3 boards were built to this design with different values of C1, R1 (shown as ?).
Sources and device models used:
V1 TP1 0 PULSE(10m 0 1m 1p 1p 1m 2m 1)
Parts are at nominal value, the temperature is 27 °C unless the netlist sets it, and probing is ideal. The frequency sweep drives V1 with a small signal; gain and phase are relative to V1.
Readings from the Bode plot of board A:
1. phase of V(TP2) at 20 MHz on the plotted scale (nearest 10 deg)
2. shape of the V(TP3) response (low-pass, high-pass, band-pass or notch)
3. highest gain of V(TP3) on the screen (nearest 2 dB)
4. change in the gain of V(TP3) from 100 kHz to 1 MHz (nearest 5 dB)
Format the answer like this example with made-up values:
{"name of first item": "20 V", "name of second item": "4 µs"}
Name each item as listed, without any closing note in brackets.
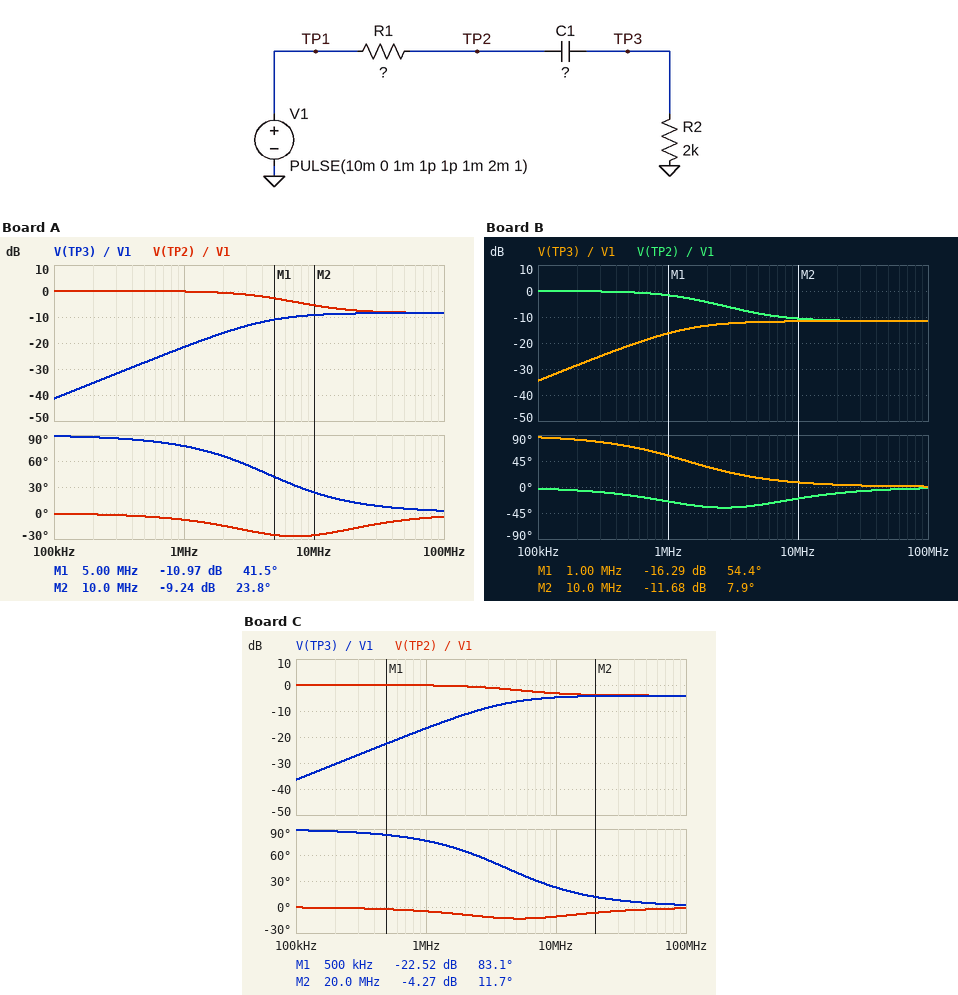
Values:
{"phase of V(TP2) at 20 MHz on the plotted scale": "-20 deg", "shape of the V(TP3) response": "high-pass", "highest gain of V(TP3) on the screen": "-8 dB", "change in the gain of V(TP3) from 100 kHz to 1 MHz": "20 dB"}
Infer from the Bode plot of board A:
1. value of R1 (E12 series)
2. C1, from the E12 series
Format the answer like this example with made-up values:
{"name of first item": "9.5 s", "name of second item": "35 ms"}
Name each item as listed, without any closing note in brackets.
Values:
{"value of R1": "3.3 kΩ", "C1, from the E12 series": "6.8 pF"}
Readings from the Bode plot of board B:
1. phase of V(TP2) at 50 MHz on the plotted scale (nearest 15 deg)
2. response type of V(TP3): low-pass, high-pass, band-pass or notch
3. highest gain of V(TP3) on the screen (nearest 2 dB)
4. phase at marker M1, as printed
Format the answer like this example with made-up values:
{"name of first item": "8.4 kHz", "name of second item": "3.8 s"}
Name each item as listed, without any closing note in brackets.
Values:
{"phase of V(TP2) at 50 MHz on the plotted scale": "0 deg", "response type of V(TP3): low-pass, high-pass, band-pass or notch": "high-pass", "highest gain of V(TP3) on the screen": "-12 dB", "phase at marker M1, as printed": "54.4 deg"}
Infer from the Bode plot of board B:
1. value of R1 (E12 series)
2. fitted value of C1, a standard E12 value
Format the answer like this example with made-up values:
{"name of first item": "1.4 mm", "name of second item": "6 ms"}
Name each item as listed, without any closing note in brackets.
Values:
{"value of R1": "5.6 kΩ", "fitted value of C1, a standard E12 value": "15 pF"}
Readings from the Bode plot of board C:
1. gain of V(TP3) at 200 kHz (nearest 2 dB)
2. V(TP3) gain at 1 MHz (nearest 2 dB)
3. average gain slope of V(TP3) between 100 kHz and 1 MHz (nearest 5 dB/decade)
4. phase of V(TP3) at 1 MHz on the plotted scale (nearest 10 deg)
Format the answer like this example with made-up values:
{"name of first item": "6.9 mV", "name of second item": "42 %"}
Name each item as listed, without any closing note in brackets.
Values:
{"gain of V(TP3) at 200 kHz": "-30 dB", "V(TP3) gain at 1 MHz": "-16 dB", "average gain slope of V(TP3) between 100 kHz and 1 MHz": "20 dB/decade", "phase of V(TP3) at 1 MHz on the plotted scale": "80 deg"}
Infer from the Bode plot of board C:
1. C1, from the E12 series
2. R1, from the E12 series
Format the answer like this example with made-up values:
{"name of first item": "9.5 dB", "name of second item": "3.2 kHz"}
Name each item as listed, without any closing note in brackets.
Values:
{"C1, from the E12 series": "12 pF", "R1, from the E12 series": "1.2 kΩ"}
